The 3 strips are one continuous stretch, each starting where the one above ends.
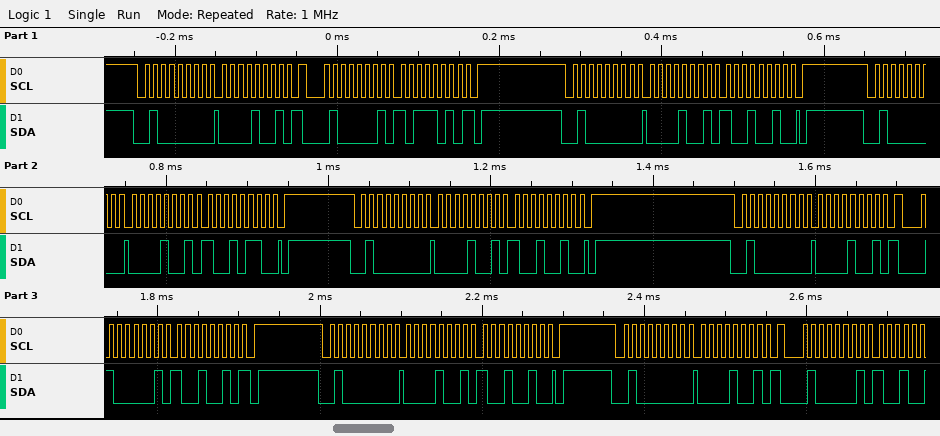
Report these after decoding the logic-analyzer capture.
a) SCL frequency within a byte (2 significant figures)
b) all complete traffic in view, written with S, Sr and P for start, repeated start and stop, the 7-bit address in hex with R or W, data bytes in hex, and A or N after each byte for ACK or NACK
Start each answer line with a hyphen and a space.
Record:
- 100 kHz
- S 20W A 09 A Sr 20R A BA N P S 20W A 09 A 92 A P S 20W A 09 A 96 A P S 20W A 09 A 92 A P S 20W A 09 A Sr 20R A 92 N P S 20W A 09 A 92 A P S 20W A 09 A Sr 20R A
